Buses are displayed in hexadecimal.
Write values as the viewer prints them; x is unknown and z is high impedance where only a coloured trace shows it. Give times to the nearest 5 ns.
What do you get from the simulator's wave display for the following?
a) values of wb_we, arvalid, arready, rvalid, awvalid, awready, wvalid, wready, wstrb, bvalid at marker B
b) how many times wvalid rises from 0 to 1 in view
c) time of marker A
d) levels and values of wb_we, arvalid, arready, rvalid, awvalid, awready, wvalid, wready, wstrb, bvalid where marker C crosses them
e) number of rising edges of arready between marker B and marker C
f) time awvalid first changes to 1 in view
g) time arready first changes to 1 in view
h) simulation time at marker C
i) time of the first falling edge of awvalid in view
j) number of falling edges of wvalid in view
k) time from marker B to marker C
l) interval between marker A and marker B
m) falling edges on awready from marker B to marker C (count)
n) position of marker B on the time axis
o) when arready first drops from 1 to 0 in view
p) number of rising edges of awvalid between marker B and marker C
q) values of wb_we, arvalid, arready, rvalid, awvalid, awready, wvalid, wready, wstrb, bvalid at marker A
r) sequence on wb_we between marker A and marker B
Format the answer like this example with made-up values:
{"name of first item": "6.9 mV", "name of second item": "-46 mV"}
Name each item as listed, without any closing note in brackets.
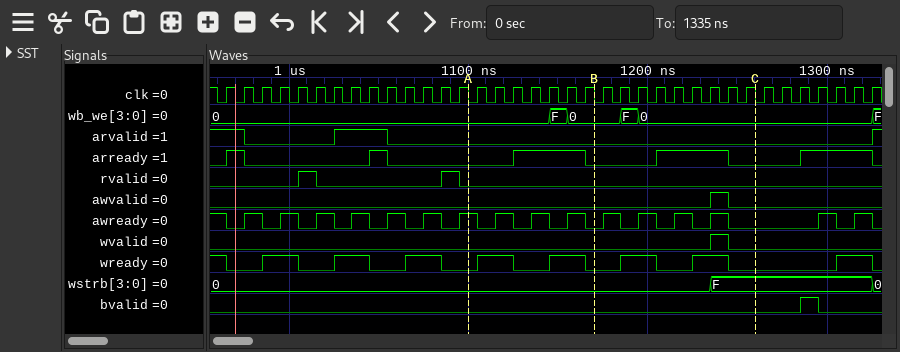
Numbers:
{"values of wb_we, arvalid, arready, rvalid, awvalid, awready, wvalid, wready, wstrb, bvalid at marker B": "wb_we=0, arvalid=0, arready=0, rvalid=0, awvalid=0, awready=0, wvalid=0, wready=0, wstrb=0, bvalid=0", "how many times wvalid rises from 0 to 1 in view": "1", "time of marker A": "1100 ns", "levels and values of wb_we, arvalid, arready, rvalid, awvalid, awready, wvalid, wready, wstrb, bvalid where marker C crosses them": "wb_we=0, arvalid=0, arready=0, rvalid=0, awvalid=0, awready=0, wvalid=0, wready=0, wstrb=F, bvalid=0", "number of rising edges of arready between marker B and marker C": "1", "time awvalid first changes to 1 in view": "1235 ns", "time arready first changes to 1 in view": "965 ns", "simulation time at marker C": "1260 ns", "time of the first falling edge of awvalid in view": "1245 ns", "number of falling edges of wvalid in view": "1", "time from marker B to marker C": "90 ns", "interval between marker A and marker B": "70 ns", "falling edges on awready from marker B to marker C": "4", "position of marker B on the time axis": "1170 ns", "when arready first drops from 1 to 0 in view": "975 ns", "number of rising edges of awvalid between marker B and marker C": "1", "values of wb_we, arvalid, arready, rvalid, awvalid, awready, wvalid, wready, wstrb, bvalid at marker A": "wb_we=0, arvalid=0, arready=0, rvalid=0, awvalid=0, awready=1, wvalid=0, wready=0, wstrb=0, bvalid=0", "sequence on wb_we between marker A and marker B": "0, F, 0"}
